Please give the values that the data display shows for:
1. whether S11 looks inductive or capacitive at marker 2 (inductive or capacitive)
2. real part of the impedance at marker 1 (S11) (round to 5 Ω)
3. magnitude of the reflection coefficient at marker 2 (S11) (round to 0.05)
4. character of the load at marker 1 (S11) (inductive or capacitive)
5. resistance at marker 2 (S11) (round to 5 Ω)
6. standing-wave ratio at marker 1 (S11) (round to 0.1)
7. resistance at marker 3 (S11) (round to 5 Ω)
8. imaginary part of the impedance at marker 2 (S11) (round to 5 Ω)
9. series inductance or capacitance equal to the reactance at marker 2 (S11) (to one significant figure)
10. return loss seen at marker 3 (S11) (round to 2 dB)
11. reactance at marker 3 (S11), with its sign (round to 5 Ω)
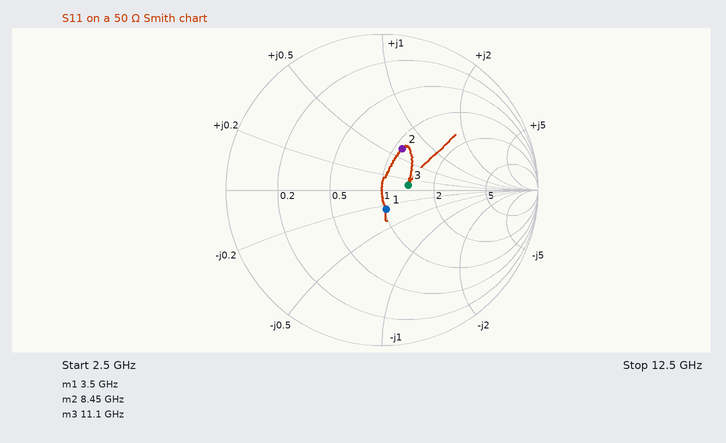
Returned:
inductive
50 Ω
0.30
capacitive
55 Ω
1.3
70 Ω
+30 Ω
600 pH
16 dB
+5 Ω
